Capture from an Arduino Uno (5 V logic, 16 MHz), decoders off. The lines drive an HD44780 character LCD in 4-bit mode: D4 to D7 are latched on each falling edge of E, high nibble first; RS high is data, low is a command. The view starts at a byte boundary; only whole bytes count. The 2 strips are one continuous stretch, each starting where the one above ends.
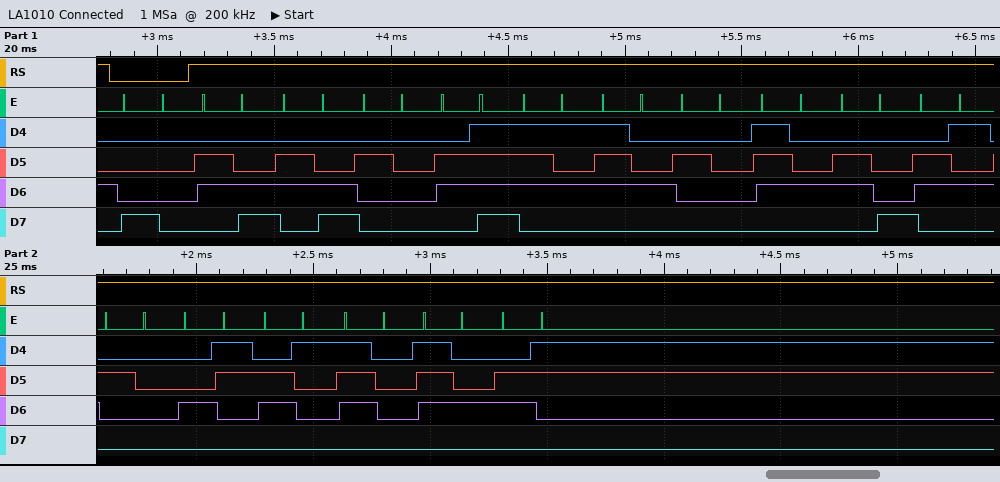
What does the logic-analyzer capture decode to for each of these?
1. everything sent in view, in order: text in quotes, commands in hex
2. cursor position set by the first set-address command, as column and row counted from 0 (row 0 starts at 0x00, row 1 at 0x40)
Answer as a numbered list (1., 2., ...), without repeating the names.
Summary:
1. 0x80 "ll out the Captc"
2. column 0, row 0
